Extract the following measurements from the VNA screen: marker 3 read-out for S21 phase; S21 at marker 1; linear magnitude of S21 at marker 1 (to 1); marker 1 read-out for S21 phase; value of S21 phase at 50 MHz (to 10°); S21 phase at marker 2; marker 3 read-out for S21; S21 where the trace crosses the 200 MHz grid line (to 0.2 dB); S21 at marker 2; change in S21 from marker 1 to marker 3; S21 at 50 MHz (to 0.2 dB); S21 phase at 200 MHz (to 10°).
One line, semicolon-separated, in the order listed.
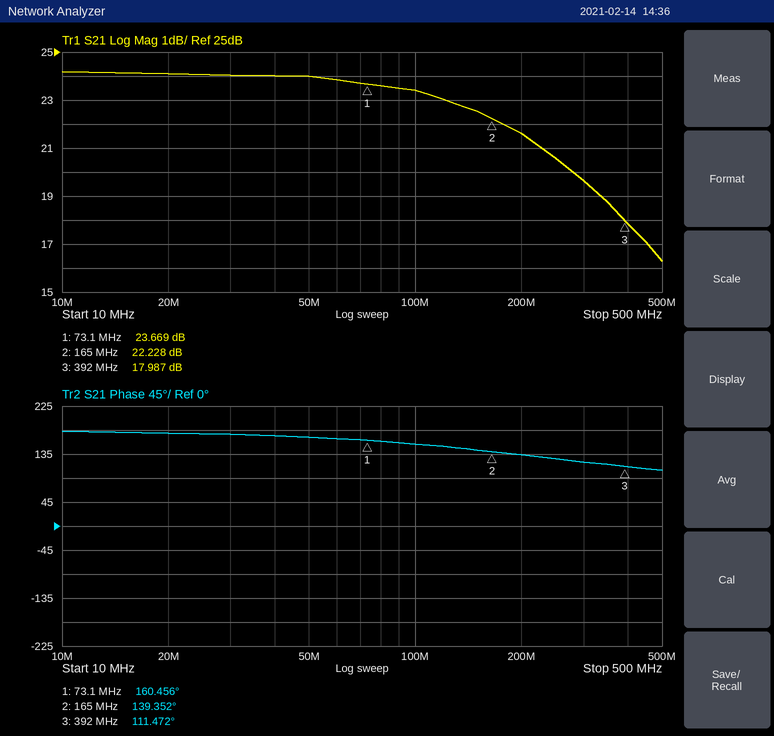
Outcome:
111.472°; 23.669 dB; 15; 160.456°; 170°; 139.352°; 17.987 dB; 21.6 dB; 22.228 dB; -5.682 dB; 24.0 dB; 130°
